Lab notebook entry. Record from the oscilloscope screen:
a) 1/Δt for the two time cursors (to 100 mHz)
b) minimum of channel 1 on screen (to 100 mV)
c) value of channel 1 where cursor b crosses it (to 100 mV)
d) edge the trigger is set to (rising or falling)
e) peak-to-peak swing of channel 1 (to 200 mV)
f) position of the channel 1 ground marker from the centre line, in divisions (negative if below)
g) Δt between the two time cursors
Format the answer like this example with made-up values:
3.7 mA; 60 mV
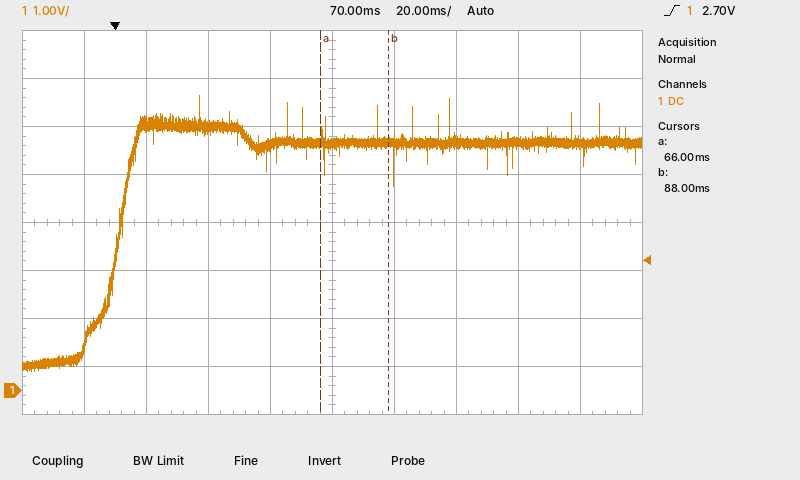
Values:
45.5 Hz; 400 mV; 5.2 V; rising; 5.8 V; -3.5 div; 22 ms
